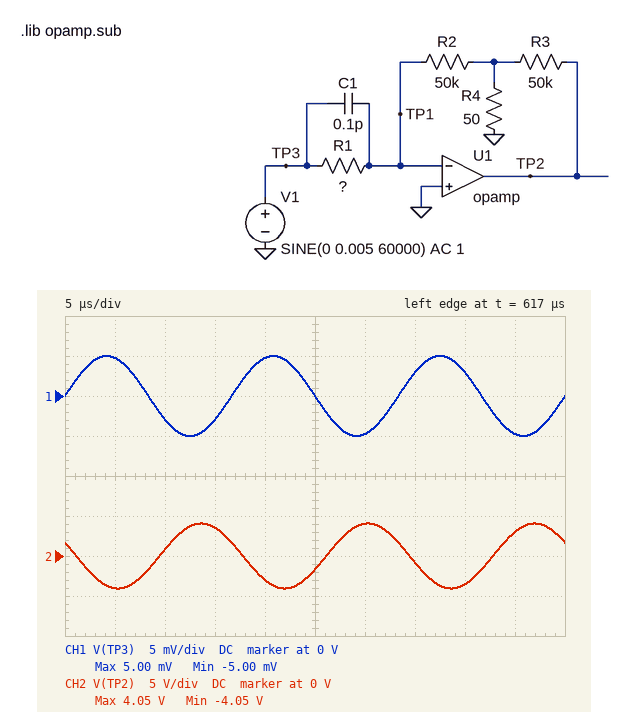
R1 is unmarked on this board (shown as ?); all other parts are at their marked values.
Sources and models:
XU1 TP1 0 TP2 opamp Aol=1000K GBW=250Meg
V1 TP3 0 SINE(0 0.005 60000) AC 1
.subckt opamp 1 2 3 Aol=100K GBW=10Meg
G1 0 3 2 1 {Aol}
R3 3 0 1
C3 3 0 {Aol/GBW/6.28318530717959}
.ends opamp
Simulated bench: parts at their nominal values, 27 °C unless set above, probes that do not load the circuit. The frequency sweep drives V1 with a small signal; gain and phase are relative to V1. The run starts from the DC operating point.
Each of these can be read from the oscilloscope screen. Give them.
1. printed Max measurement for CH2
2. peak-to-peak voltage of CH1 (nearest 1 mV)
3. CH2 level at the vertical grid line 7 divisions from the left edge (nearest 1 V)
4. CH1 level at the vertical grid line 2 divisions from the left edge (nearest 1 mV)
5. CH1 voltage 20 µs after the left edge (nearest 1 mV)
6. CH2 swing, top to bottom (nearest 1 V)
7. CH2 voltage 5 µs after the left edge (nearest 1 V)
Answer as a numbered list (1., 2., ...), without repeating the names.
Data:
1. 4.05 V
2. 10 mV
3. -1 V
4. -3 mV
5. 5 mV
6. 8 V
7. -4 V
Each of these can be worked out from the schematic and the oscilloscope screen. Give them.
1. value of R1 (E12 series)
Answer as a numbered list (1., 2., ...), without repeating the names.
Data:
1. 56 kΩ
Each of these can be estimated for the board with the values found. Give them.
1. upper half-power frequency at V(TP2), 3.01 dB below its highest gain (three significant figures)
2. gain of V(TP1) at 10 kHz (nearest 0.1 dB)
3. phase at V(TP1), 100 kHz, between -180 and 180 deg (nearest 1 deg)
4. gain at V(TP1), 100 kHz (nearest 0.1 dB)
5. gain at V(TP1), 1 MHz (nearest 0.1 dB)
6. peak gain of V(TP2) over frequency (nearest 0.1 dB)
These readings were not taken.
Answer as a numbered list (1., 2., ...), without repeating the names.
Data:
1. 132 kHz
2. -29.0 dB
3. 53 deg
4. -10.9 dB
5. -6.6 dB
6. 59.0 dB
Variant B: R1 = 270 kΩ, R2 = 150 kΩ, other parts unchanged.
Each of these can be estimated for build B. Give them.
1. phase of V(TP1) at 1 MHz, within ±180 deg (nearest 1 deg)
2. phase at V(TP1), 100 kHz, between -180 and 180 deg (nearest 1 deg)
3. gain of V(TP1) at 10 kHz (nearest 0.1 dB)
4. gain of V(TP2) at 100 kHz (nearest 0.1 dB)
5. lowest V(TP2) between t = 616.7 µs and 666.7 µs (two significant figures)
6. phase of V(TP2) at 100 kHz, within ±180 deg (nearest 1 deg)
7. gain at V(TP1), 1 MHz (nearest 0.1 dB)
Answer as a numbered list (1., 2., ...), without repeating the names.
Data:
1. 15 deg
2. 59 deg
3. -33.1 dB
4. 53.5 dB
5. -2.6 V
6. 149 deg
7. -8.9 dB
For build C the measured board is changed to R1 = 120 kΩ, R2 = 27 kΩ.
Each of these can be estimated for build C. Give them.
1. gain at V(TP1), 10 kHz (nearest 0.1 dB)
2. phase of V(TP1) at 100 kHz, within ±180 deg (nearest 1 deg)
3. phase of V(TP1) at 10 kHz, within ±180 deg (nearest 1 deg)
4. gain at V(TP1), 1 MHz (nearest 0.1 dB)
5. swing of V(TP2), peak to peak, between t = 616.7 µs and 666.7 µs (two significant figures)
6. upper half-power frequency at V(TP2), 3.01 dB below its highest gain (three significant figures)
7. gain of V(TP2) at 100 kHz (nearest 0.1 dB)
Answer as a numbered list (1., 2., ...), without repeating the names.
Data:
1. -40.9 dB
2. 64 deg
3. 86 deg
4. -14.8 dB
5. 2.2 V
6. 205 kHz
7. 46.1 dB
